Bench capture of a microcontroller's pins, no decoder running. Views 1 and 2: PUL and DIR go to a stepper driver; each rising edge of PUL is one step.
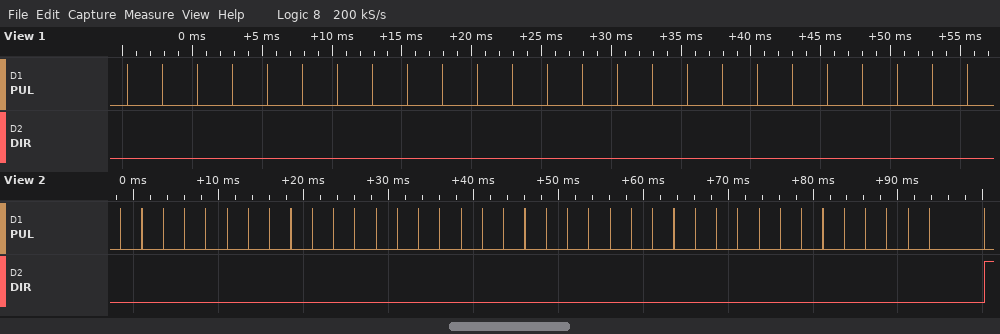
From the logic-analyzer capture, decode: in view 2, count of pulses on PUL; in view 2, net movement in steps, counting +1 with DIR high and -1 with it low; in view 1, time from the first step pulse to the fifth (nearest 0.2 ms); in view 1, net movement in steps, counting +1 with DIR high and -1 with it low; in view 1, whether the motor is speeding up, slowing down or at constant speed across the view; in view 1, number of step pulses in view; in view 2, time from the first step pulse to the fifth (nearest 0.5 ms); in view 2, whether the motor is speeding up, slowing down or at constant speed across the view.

40
-38
10.0 ms
-25
constant speed
25
10.0 ms
slowing down
